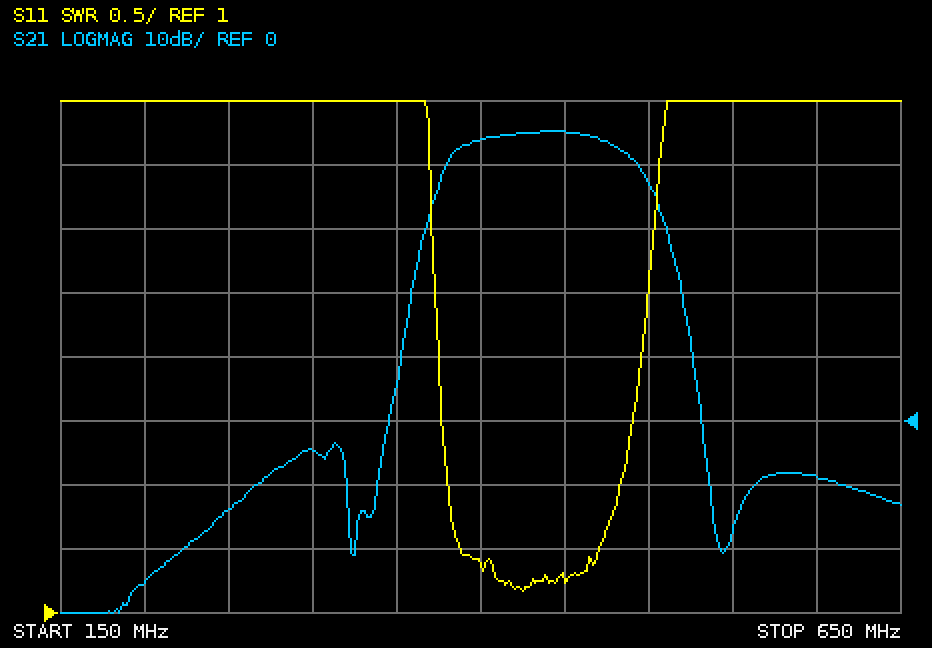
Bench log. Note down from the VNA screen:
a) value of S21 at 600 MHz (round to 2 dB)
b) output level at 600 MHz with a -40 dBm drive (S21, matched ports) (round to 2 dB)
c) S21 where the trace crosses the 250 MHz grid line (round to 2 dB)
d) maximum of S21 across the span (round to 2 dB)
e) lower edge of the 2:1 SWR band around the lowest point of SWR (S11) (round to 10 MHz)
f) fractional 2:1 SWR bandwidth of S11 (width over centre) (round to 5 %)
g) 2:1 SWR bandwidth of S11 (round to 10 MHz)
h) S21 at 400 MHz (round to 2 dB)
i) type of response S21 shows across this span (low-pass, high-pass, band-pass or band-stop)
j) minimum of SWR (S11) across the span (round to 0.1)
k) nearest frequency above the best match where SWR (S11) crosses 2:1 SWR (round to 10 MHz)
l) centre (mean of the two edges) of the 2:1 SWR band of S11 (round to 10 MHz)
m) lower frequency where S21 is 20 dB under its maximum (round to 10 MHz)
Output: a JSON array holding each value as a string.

["-8 dB", "-48 dBm", "-14 dB", "46 dB", "380 MHz", "25 %", "100 MHz", "44 dB", "band-pass", "1.2", "480 MHz", "430 MHz", "360 MHz"]
